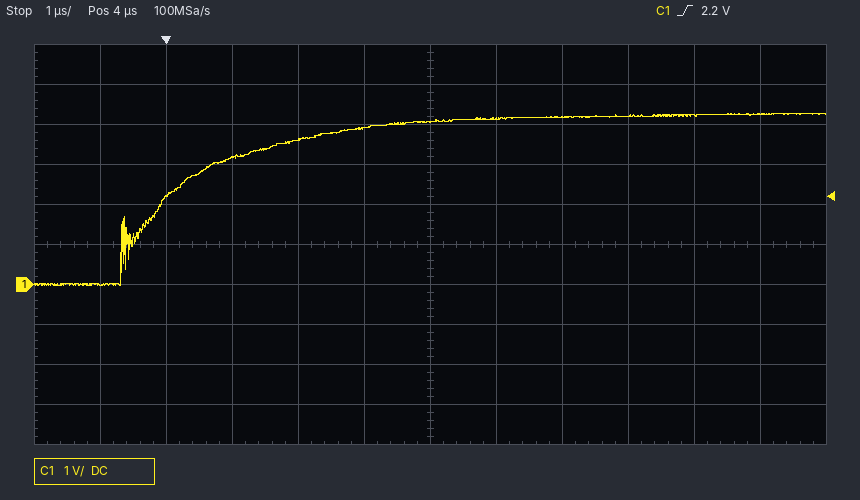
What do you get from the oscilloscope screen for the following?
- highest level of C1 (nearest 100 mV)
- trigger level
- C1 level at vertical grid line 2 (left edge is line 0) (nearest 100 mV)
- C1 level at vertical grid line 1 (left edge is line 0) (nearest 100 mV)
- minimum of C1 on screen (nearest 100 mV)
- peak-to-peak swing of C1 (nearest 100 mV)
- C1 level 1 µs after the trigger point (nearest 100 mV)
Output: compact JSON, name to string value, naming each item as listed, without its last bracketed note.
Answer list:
{"highest level of C1": "4.3 V", "trigger level": "2.2 V", "C1 level at vertical grid line 2 (left edge is line 0)": "2.2 V", "C1 level at vertical grid line 1 (left edge is line 0)": "0.0 V", "minimum of C1 on screen": "0.0 V", "peak-to-peak swing of C1": "4.3 V", "C1 level 1 µs after the trigger point": "3.2 V"}
